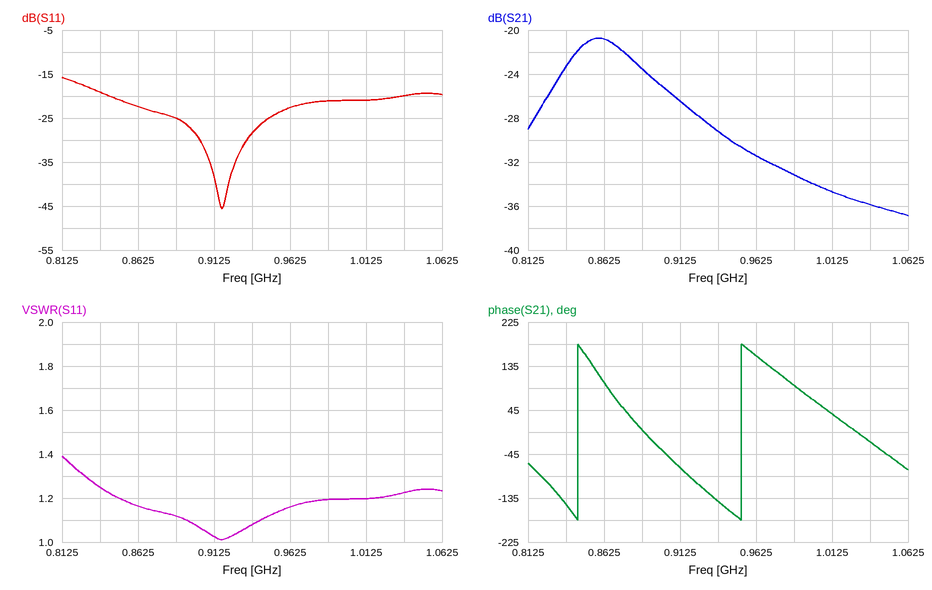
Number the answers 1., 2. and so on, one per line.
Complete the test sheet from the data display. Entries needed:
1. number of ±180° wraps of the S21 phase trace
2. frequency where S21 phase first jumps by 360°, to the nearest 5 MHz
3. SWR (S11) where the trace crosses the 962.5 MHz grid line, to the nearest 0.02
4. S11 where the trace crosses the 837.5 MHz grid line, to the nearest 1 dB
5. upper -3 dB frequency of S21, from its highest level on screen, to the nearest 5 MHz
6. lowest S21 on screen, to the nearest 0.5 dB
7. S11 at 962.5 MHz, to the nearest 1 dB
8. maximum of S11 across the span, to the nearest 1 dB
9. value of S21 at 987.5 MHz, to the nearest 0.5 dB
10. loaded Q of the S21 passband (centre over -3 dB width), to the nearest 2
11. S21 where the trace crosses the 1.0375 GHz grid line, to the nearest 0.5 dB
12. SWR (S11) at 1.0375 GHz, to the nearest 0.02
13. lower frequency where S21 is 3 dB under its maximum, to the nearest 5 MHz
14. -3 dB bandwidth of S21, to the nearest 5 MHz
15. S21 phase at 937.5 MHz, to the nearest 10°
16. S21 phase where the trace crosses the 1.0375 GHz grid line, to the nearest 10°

1. 2
2. 845 MHz
3. 1.16
4. -19 dB
5. 890 MHz
6. -37.0 dB
7. -23 dB
8. -16 dB
9. -33.0 dB
10. 16
11. -36.0 dB
12. 1.22
13. 835 MHz
14. 55 MHz
15. -140°
16. -20°
